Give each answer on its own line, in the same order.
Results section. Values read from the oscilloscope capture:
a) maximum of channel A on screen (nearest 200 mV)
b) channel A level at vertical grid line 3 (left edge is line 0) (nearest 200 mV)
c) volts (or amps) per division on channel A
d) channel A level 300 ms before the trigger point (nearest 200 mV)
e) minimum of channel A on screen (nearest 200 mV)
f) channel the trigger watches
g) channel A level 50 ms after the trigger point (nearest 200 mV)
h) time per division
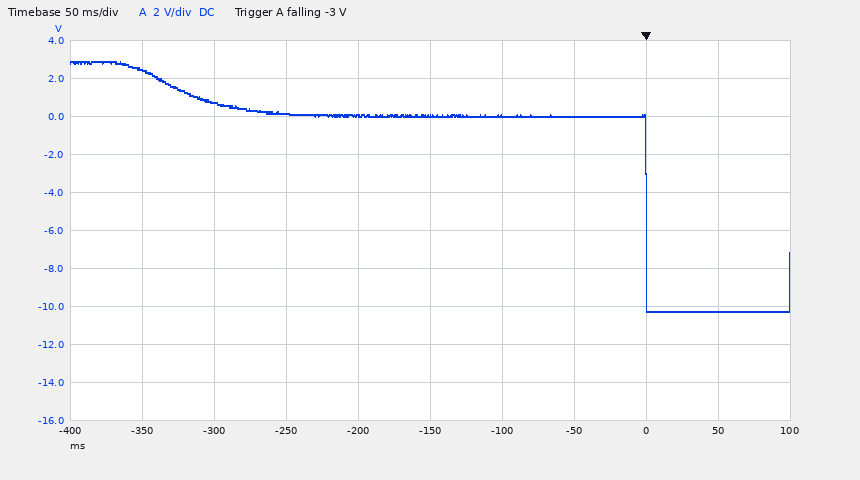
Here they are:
2.8 V
200 mV
2 V
800 mV
-10.2 V
channel A
-10.2 V
50 ms
